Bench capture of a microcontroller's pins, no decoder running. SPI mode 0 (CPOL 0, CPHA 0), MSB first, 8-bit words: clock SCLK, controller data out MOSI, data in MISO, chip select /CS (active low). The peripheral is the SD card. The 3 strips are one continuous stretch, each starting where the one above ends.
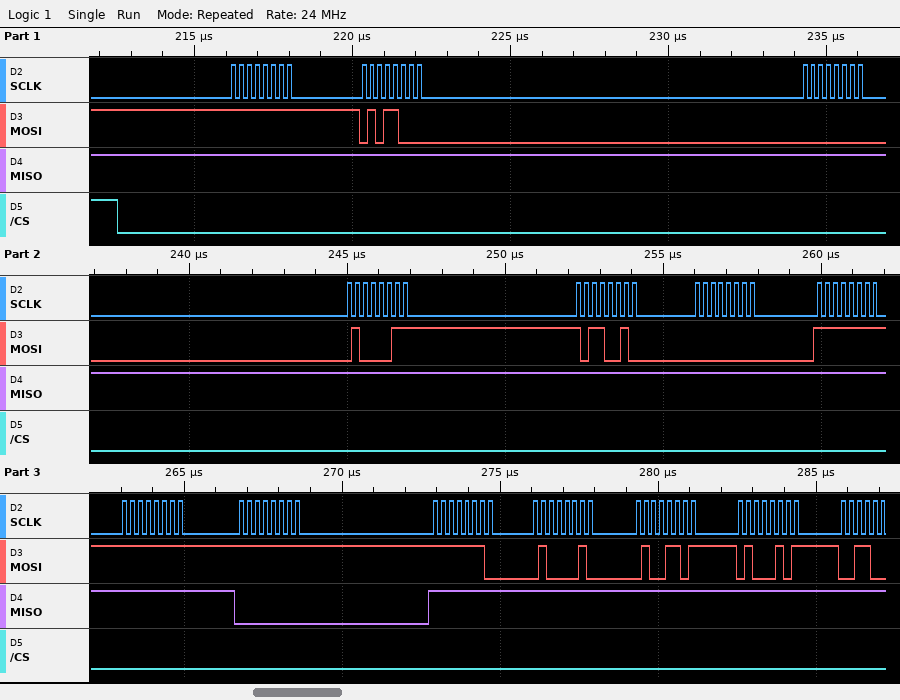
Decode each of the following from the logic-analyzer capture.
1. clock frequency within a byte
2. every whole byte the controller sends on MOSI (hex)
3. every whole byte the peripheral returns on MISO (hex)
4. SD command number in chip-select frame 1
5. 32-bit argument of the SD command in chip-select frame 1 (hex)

4 MHz
FF 58 00 43 B2 00 FF FF FF FE 42 4D 45
FF FF FF FF FF FF FF FF 00 FF FF FF FF
CMD24
0x0043B200
